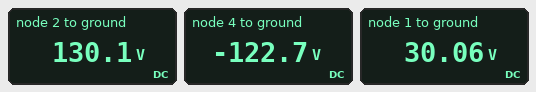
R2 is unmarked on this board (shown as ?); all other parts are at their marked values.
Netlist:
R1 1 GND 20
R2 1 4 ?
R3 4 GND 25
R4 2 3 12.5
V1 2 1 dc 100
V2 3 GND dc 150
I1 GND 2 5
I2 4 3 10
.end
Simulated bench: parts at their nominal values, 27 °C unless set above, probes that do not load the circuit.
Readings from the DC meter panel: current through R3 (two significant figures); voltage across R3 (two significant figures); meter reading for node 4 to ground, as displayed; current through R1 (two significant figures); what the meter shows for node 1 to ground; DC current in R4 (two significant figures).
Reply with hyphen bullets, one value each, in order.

- 4.9 A
- 120 V
- -122.7 V
- 1.5 A
- 30.06 V
- 1.6 A
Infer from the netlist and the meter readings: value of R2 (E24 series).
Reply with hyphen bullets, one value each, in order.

- 30 Ω
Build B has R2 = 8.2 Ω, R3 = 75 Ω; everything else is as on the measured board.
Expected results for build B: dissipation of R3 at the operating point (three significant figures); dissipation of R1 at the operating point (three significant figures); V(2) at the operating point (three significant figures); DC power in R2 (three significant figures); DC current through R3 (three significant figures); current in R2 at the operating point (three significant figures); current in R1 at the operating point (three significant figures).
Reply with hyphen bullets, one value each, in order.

- 73.0 W
- 516 µW
- 99.9 V
- 666 W
- 987 mA
- 9.01 A
- 5.08 mA
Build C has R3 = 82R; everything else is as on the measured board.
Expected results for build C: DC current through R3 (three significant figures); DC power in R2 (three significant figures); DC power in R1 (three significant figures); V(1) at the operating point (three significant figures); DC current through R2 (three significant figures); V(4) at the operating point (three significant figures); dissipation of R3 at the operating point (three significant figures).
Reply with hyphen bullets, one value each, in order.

- 2.57 A
- 1.66 kW
- 7.30 W
- 12.1 V
- 7.43 A
- -211 V
- 542 W
